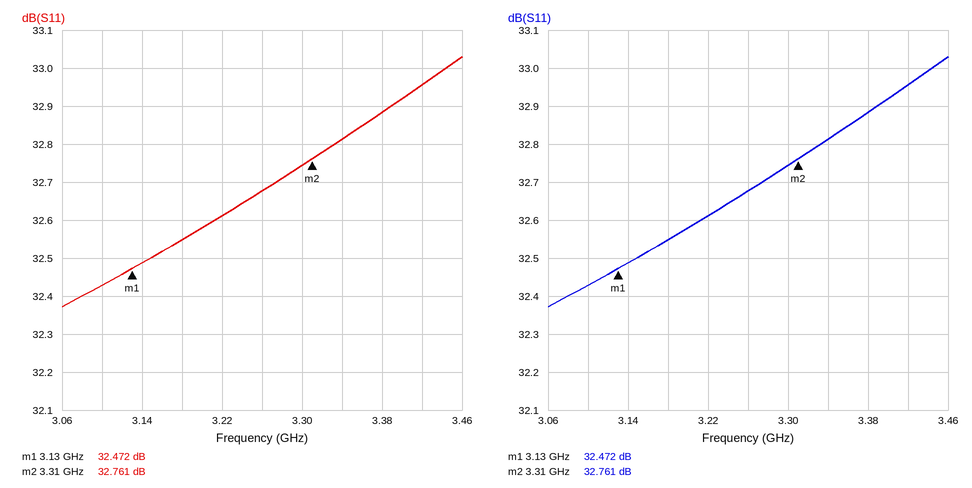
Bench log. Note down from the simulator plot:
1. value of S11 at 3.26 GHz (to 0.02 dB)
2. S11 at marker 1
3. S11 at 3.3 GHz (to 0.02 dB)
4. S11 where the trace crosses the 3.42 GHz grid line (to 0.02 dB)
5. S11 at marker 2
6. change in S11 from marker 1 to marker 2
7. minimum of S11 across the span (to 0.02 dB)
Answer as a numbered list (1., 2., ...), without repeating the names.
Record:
1. 32.68 dB
2. 32.472 dB
3. 32.74 dB
4. 32.96 dB
5. 32.761 dB
6. 0.289 dB
7. 32.38 dB
